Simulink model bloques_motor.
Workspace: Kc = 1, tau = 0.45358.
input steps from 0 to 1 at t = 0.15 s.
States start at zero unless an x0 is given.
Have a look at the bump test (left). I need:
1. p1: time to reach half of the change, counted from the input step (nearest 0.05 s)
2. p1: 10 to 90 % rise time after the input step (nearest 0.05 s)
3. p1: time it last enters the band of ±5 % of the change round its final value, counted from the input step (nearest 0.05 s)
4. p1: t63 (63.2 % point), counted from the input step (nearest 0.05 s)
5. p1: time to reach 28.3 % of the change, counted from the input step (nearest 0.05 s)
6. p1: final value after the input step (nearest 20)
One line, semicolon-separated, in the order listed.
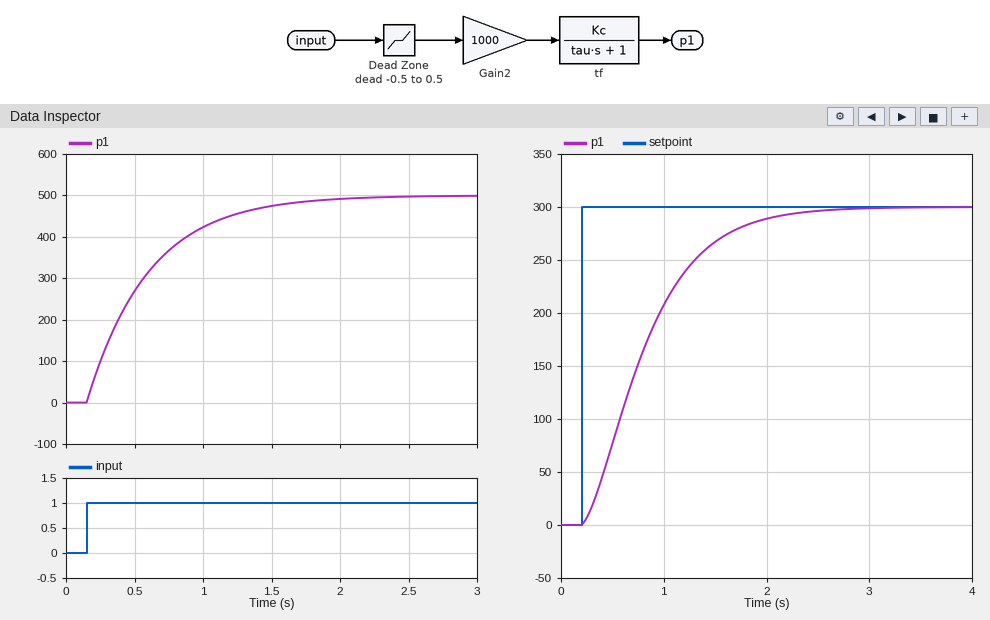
0.30 s; 1.00 s; 1.35 s; 0.45 s; 0.15 s; 500
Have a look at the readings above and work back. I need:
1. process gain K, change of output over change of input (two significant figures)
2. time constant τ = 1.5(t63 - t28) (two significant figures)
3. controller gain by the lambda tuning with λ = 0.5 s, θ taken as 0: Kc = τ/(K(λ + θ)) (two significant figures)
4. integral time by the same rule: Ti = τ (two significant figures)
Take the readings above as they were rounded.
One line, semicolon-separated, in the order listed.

500; 0.45 s; 0.0018; 0.45 s
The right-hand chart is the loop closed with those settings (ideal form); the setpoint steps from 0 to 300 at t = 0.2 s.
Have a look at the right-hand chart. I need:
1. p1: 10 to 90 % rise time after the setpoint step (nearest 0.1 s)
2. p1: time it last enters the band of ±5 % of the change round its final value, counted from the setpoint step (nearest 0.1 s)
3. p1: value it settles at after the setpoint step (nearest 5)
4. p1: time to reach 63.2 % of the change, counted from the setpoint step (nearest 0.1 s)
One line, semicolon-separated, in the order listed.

1.2 s; 1.7 s; 300; 0.7 s
